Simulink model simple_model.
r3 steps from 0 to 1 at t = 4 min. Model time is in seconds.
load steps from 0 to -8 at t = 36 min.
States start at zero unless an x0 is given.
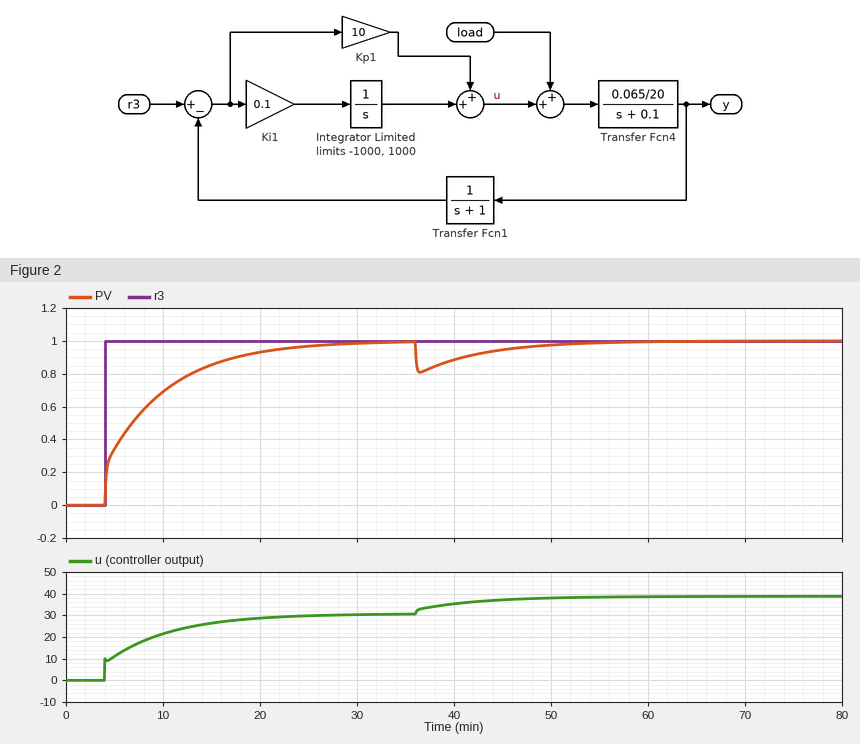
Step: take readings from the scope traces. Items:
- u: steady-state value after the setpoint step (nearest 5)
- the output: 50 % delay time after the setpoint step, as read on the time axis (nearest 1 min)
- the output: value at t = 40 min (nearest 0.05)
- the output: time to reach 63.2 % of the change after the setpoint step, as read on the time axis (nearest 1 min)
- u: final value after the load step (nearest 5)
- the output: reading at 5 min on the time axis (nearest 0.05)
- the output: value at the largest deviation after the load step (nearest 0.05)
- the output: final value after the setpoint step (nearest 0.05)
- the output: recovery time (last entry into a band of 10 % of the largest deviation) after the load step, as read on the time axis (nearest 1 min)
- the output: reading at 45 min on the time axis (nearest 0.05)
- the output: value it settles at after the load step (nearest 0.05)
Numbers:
30
7 min
0.90
9 min
40
0.35
0.80
1.00
52 min
0.95
1.00
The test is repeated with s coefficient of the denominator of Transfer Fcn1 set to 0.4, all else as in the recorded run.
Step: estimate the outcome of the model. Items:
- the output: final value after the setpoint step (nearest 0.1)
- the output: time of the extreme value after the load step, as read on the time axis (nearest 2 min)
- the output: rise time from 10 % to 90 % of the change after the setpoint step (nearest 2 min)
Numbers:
1.0
36 min
14 min
